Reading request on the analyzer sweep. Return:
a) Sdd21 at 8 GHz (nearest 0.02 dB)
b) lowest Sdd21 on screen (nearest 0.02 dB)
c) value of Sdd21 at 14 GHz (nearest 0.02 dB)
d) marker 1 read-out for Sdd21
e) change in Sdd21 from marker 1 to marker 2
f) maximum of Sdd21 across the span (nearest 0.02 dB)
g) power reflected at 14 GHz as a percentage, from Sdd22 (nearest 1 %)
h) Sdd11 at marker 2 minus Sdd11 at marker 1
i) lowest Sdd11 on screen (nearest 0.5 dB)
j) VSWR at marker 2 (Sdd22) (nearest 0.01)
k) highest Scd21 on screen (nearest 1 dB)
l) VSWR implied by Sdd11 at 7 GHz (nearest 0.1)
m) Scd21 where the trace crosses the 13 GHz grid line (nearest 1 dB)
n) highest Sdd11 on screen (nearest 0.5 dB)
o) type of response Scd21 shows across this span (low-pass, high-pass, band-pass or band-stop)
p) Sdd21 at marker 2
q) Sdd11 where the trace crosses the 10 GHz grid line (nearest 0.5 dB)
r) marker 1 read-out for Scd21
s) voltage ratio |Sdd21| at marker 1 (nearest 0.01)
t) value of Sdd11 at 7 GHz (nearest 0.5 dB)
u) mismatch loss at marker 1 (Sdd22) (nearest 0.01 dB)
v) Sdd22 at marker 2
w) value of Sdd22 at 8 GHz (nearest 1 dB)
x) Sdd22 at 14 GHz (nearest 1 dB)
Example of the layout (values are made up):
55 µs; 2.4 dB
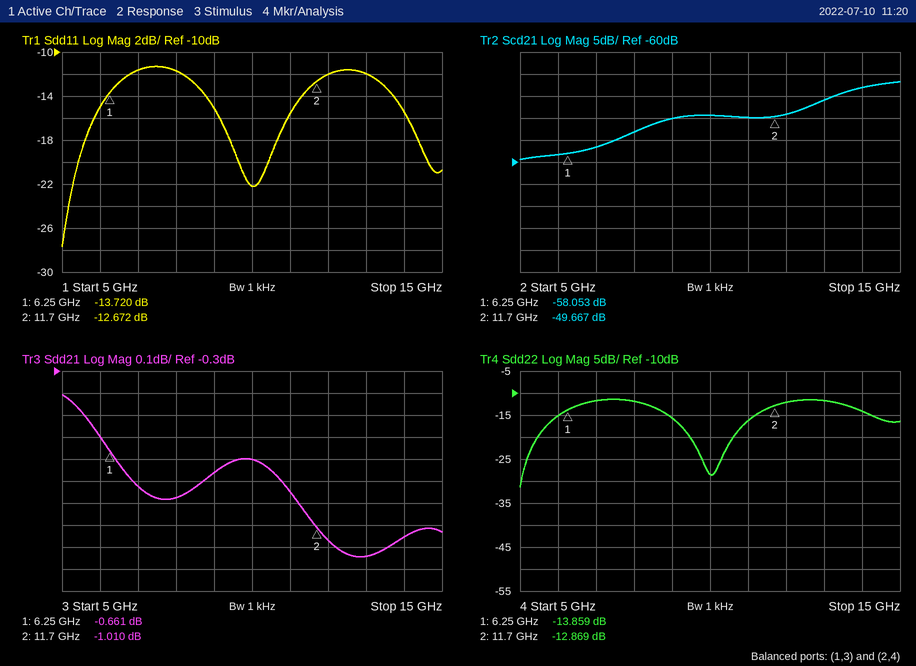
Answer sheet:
-0.88 dB; -1.14 dB; -1.06 dB; -0.661 dB; -0.349 dB; -0.40 dB; 4 %; 1.048 dB; -27.5 dB; 1.59; -42 dB; 1.7; -46 dB; -11.5 dB; high-pass; -1.010 dB; -22.0 dB; -58.053 dB; 0.93; -11.5 dB; 0.18 dB; -12.869 dB; -12 dB; -14 dB
